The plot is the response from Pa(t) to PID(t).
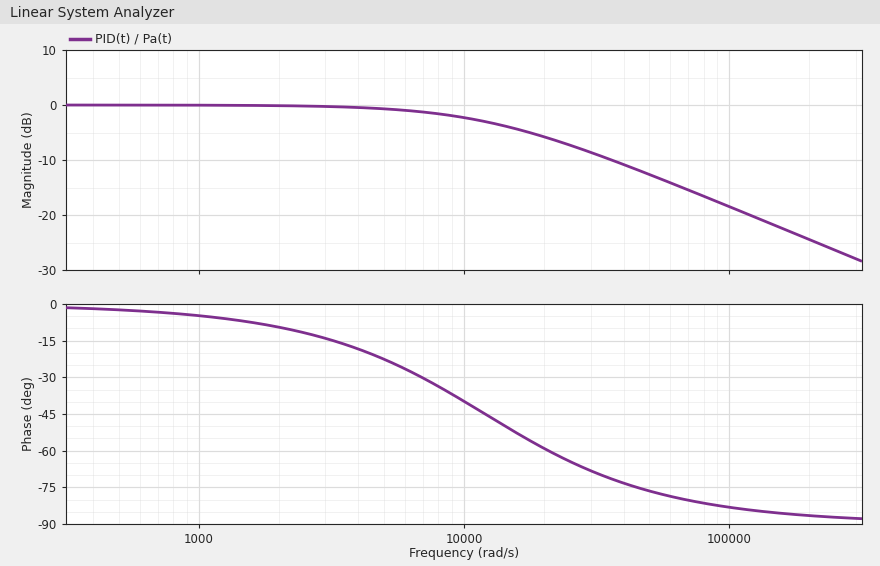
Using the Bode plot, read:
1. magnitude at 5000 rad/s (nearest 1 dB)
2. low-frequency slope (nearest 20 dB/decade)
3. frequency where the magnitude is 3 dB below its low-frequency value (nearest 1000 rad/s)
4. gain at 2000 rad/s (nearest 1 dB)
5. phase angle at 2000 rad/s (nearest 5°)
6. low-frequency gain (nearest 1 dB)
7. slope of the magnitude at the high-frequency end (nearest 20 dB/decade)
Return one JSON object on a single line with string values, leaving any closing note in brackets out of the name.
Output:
{"magnitude at 5000 rad/s": "-1 dB", "low-frequency slope": "0 dB/decade", "frequency where the magnitude is 3 dB below its low-frequency value": "12000 rad/s", "gain at 2000 rad/s": "0 dB", "phase angle at 2000 rad/s": "-10°", "low-frequency gain": "0 dB", "slope of the magnitude at the high-frequency end": "-20 dB/decade"}
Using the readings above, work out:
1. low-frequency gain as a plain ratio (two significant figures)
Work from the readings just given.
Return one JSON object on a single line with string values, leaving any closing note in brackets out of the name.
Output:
{"low-frequency gain as a plain ratio": "1.0"}
